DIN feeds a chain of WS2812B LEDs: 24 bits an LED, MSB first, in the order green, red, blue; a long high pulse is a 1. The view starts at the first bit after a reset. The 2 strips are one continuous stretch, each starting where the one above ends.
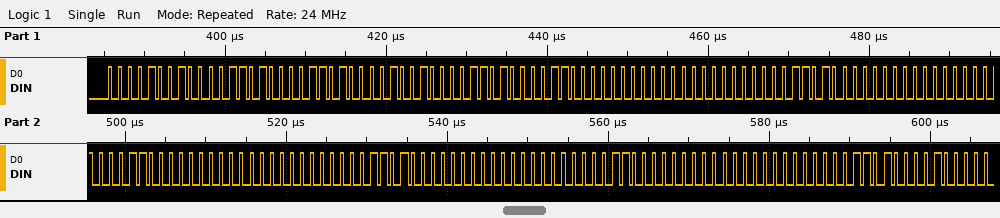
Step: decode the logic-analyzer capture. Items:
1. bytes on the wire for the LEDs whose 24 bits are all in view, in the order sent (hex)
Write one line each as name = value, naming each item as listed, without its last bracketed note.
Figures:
bytes on the wire for the LEDs whose 24 bits are all in view, in the order sent = 09 0D 0D 09 0D 0C 00 00 0D 00 00 0C 00 00 0D 00 00 0C 00 00 0D
